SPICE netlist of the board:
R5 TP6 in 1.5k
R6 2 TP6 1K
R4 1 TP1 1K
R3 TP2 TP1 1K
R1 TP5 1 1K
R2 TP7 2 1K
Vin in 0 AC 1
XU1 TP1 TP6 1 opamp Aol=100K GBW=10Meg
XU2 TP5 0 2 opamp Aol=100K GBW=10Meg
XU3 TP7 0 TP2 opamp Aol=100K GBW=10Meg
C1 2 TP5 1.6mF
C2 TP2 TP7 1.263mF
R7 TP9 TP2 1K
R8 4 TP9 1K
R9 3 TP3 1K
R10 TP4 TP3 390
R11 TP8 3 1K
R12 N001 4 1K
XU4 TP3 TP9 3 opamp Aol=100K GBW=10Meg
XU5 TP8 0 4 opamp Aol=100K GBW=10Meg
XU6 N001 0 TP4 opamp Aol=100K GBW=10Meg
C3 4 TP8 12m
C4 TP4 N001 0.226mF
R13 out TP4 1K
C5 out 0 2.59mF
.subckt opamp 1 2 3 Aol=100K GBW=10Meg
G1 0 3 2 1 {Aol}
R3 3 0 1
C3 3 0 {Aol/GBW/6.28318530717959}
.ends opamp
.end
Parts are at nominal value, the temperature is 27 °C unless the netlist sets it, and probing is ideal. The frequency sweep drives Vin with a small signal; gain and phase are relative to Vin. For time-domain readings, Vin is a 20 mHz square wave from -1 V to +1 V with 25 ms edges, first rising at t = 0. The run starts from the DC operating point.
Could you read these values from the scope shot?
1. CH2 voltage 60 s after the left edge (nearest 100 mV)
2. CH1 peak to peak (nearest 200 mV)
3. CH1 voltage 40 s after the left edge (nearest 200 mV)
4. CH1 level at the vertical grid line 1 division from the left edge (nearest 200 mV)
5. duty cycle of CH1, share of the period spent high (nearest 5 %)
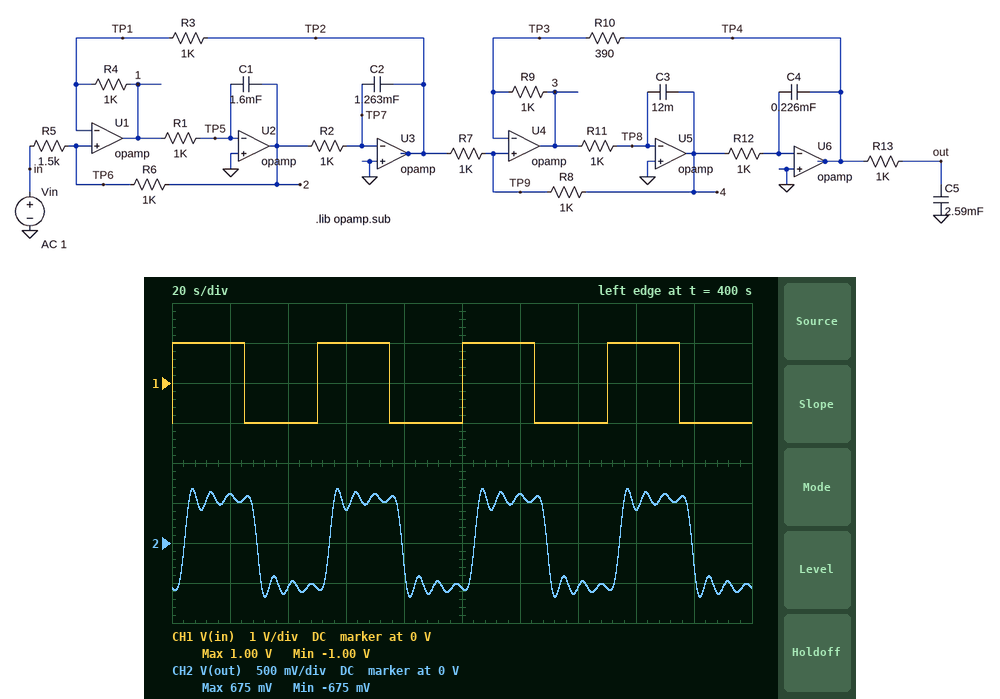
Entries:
400 mV
2.0 V
-1.0 V
1.0 V
50 %
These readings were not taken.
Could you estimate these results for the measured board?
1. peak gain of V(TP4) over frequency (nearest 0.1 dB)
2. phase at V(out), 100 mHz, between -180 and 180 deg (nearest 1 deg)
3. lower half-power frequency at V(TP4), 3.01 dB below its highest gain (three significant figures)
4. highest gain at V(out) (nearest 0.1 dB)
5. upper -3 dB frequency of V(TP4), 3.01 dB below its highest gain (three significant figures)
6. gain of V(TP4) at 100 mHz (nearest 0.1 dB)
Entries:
6.7 dB
-146 deg
136 mHz
-1.8 dB
163 mHz
-0.3 dB
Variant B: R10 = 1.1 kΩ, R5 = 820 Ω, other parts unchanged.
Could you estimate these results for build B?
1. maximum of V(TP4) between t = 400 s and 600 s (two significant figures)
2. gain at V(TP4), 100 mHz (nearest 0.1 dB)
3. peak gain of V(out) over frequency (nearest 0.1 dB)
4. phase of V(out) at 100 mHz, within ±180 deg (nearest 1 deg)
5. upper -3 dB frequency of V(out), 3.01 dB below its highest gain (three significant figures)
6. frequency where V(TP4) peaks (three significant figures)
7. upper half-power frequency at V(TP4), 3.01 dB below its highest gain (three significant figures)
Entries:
3.6 V
16.5 dB
16.1 dB
87 deg
97.3 mHz
91.7 mHz
97.8 mHz
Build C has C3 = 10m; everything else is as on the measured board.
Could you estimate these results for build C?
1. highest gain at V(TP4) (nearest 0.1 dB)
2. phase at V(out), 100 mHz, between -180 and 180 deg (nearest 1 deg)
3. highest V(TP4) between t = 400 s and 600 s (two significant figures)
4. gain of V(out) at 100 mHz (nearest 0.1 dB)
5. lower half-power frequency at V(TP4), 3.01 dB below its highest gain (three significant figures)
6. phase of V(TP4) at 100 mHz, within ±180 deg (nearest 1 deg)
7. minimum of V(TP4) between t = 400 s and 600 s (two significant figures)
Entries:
4.4 dB
-145 deg
1.1 V
-6.9 dB
144 mHz
-87 deg
-1.1 V
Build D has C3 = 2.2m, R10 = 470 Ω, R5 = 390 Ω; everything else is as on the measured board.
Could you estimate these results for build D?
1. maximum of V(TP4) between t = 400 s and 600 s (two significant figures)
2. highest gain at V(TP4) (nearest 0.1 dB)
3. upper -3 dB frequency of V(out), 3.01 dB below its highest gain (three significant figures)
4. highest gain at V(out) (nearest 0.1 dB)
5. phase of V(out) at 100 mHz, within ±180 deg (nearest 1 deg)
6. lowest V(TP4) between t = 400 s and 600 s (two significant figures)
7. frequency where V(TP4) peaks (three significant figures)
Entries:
2.1 V
7.7 dB
125 mHz
1.9 dB
-131 deg
-2.1 V
106 mHz
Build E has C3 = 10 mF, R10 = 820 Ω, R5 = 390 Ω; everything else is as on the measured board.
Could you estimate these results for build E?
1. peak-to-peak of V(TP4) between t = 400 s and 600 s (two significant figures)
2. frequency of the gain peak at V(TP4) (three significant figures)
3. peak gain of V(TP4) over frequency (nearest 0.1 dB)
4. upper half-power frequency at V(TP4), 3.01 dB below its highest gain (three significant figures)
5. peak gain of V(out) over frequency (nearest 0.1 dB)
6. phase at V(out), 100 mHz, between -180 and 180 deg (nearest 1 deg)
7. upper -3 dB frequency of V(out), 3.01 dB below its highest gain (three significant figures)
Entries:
8.3 V
115 mHz
24.5 dB
123 mHz
17.9 dB
-150 deg
122 mHz
